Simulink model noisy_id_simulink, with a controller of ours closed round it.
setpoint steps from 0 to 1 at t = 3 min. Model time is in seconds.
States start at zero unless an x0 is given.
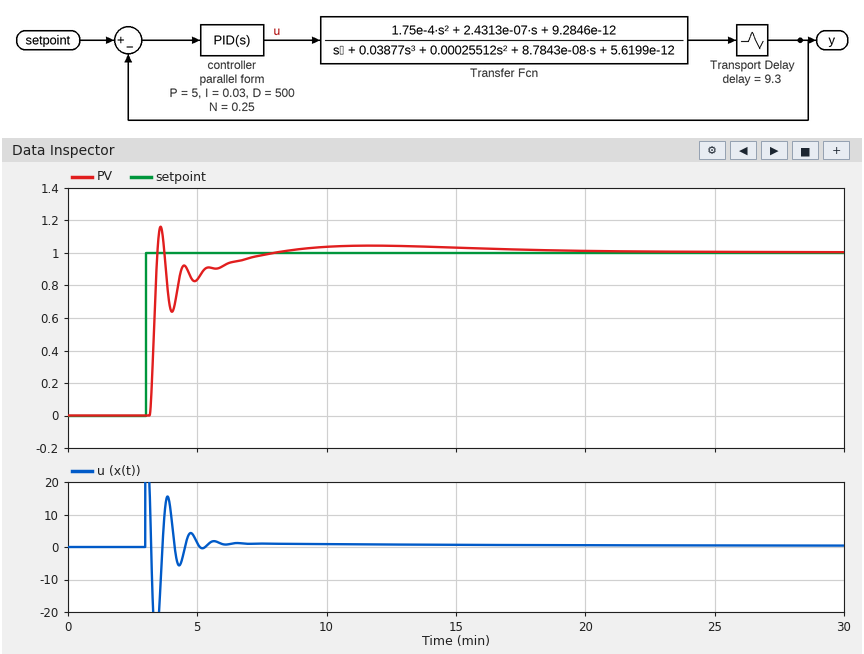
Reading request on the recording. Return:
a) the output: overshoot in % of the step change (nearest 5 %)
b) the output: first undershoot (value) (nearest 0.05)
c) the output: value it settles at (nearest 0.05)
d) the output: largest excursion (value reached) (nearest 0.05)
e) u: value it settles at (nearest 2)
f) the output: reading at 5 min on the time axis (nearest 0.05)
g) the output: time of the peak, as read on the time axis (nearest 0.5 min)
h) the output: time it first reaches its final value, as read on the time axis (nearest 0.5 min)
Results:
15 %
0.65
1.00
1.15
0
0.85
3.5 min
3.5 min
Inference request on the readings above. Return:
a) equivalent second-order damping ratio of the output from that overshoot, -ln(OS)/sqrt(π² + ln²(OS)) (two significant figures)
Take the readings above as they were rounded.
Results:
0.52
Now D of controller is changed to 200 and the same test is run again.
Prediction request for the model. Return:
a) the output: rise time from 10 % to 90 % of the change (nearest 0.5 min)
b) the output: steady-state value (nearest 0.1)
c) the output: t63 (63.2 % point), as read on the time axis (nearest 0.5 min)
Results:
1.5 min
1.0
3.5 min
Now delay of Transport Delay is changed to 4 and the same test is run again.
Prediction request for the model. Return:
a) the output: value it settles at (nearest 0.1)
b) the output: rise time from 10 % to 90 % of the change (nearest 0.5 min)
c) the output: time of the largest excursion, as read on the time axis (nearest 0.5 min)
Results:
1.0
2.5 min
12.0 min
